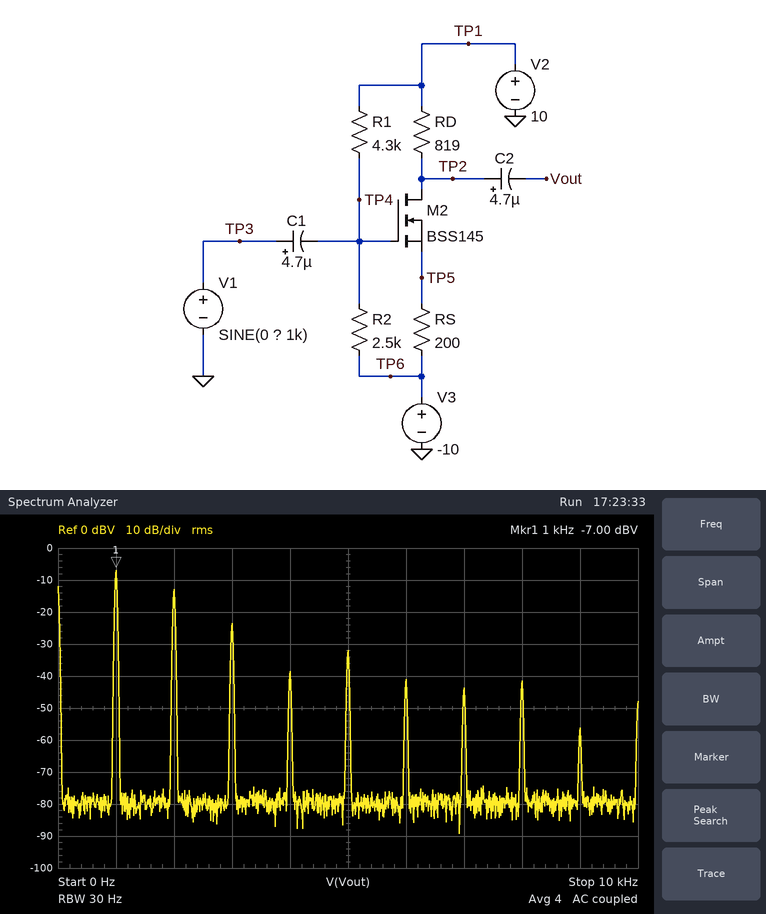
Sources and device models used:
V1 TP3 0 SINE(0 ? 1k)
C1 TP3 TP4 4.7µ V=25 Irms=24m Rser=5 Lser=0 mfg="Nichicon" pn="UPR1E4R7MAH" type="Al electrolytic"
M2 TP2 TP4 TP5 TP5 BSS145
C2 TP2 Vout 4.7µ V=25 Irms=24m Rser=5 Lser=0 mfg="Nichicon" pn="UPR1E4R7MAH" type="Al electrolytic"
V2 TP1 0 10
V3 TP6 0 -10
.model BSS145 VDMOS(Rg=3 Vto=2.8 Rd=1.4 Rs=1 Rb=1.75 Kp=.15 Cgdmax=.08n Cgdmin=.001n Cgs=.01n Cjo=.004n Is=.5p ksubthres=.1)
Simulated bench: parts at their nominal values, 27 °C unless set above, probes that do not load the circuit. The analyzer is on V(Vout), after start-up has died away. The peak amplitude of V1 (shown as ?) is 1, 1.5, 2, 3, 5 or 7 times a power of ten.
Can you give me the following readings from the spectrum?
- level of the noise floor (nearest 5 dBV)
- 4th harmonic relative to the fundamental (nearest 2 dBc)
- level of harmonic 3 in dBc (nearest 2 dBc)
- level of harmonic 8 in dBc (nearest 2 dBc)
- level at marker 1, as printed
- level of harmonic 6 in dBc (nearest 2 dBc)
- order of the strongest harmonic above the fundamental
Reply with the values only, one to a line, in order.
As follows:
-80 dBV
-32 dBc
-16 dBc
-34 dBc
-7.00 dBV
-34 dBc
2
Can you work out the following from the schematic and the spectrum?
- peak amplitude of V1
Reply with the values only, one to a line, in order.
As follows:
500 mV
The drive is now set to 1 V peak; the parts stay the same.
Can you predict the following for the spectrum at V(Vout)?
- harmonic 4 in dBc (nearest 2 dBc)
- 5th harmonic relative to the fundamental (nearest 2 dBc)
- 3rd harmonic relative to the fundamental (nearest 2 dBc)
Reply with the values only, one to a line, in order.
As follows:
-22 dBc
-28 dBc
-24 dBc
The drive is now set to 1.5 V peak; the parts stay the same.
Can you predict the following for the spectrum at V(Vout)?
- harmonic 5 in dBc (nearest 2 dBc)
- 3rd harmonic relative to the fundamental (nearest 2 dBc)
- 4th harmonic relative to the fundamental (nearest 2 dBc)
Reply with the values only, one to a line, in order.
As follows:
-32 dBc
-28 dBc
-22 dBc
